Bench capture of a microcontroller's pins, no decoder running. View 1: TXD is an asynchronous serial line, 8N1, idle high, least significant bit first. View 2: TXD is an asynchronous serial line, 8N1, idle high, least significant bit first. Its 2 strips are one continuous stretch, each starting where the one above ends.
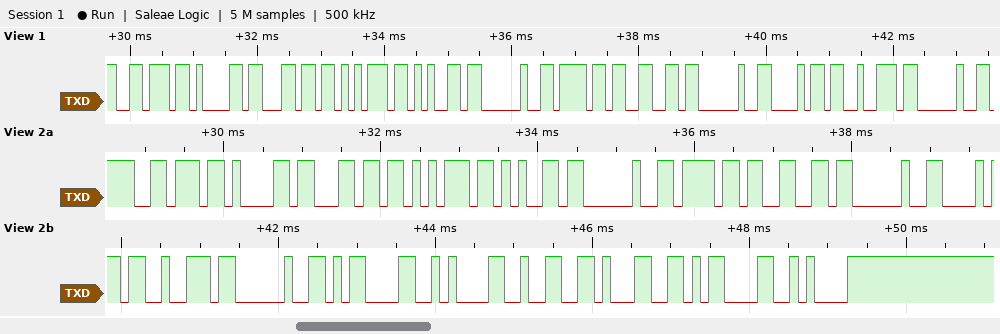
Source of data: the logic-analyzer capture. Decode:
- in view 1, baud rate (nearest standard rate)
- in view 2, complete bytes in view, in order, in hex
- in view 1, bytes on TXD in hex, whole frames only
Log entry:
9600 baud
76 61 6C 75 65 20 6F 66 20 68 72 20 0D 0A 32 31 0D 0A
76 61 6C 75 65 20 6F 66 20 68 72 20
